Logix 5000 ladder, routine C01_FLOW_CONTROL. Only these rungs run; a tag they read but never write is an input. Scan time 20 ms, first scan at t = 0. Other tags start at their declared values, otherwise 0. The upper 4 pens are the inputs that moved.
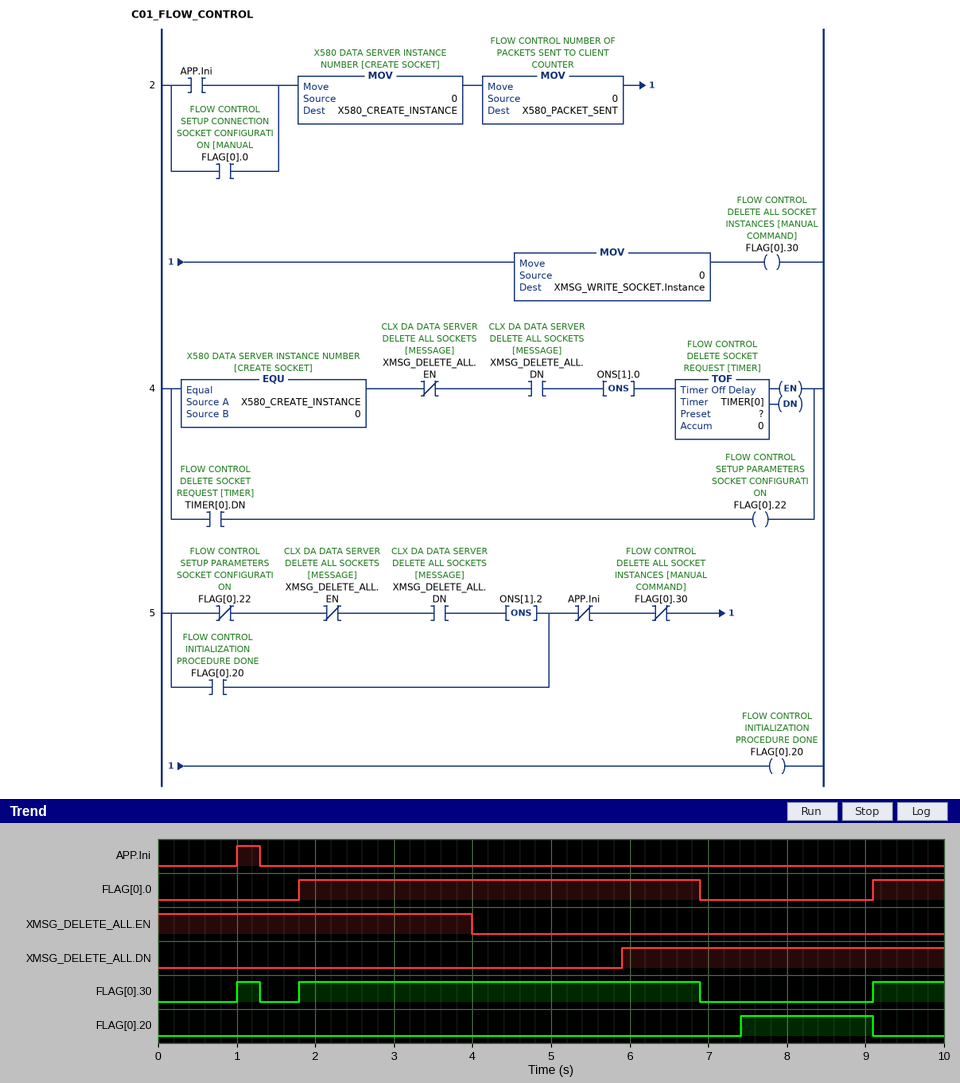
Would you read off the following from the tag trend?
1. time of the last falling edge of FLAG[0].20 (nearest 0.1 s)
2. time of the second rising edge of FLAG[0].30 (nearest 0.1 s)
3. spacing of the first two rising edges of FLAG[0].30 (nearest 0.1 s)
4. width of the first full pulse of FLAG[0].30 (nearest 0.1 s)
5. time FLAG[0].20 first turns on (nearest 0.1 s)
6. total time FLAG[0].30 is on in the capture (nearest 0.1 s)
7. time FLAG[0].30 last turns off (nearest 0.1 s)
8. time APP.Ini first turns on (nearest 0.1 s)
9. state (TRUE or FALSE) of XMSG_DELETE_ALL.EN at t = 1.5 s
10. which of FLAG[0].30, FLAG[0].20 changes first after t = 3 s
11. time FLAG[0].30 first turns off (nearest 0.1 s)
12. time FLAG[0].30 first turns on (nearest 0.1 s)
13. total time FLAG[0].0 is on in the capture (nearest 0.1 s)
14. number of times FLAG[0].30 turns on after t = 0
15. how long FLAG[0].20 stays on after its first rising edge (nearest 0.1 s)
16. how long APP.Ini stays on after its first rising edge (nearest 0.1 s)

9.1 s
1.8 s
0.8 s
0.3 s
7.4 s
6.3 s
6.9 s
1.0 s
TRUE
FLAG[0].30
1.3 s
1.0 s
6.0 s
3
1.7 s
0.3 s
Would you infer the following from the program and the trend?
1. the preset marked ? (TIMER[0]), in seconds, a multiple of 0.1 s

1.5 s
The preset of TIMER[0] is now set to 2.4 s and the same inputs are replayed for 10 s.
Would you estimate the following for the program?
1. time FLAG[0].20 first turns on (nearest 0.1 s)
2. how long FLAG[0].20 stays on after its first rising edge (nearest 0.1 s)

8.3 s
0.8 s
